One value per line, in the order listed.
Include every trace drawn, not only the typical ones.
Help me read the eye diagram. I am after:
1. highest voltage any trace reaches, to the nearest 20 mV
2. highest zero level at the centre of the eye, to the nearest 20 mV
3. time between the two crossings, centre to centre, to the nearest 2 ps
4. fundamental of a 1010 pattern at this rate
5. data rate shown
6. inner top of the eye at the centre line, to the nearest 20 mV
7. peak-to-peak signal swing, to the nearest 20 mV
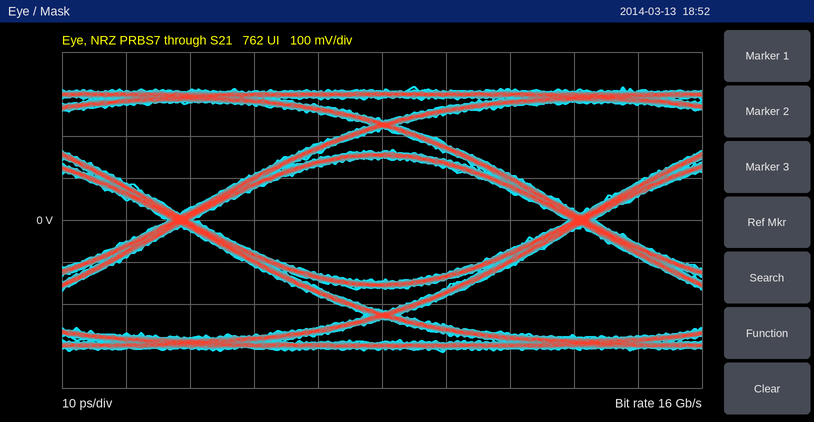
320 mV
-140 mV
62 ps
8 GHz
16 Gb/s
140 mV
640 mV
